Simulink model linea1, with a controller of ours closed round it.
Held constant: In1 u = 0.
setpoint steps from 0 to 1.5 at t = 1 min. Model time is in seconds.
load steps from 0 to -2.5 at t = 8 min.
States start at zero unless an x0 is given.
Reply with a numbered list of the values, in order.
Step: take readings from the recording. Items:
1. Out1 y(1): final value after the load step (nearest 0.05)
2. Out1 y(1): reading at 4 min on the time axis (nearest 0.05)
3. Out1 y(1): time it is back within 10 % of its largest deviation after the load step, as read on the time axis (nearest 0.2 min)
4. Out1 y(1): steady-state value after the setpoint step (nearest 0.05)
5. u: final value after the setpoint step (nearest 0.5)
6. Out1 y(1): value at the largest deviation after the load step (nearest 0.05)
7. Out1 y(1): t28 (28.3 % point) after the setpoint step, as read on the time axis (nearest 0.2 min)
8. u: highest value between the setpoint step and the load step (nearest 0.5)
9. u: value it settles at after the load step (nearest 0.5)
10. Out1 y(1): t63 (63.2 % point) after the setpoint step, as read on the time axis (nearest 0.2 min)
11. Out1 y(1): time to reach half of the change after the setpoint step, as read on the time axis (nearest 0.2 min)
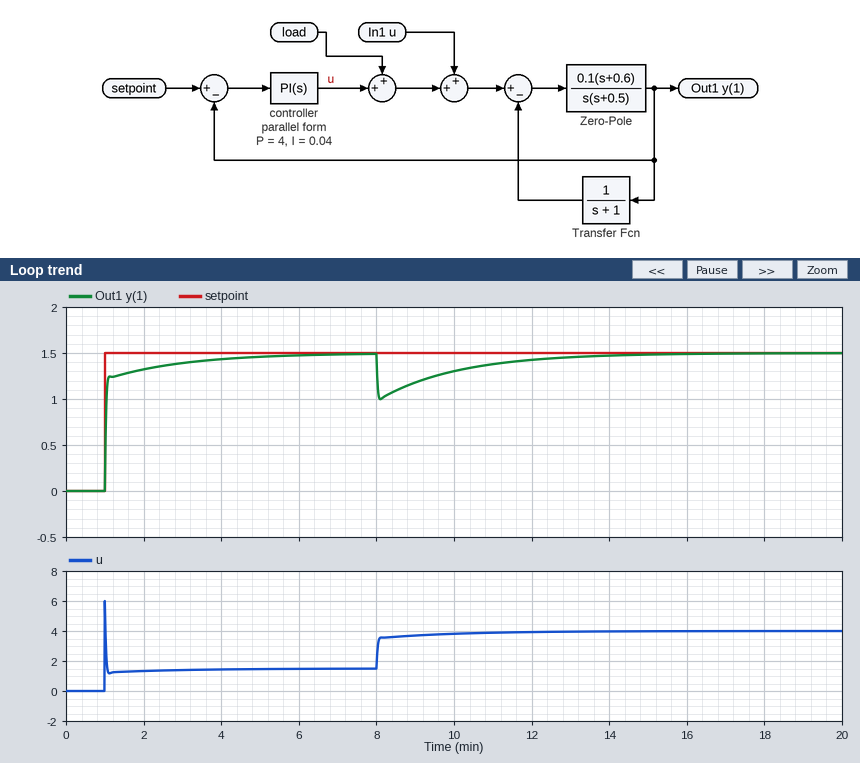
1. 1.50
2. 1.45
3. 12.8 min
4. 1.50
5. 1.5
6. 1.00
7. 1.0 min
8. 6.0
9. 4.0
10. 1.0 min
11. 1.0 min
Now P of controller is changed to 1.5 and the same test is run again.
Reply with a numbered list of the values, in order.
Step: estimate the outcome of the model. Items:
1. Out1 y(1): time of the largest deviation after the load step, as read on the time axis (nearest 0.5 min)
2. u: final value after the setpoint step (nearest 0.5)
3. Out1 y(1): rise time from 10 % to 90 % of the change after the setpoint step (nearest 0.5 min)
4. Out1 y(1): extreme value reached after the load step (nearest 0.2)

1. 8.0 min
2. 1.5
3. 1.5 min
4. 0.6
